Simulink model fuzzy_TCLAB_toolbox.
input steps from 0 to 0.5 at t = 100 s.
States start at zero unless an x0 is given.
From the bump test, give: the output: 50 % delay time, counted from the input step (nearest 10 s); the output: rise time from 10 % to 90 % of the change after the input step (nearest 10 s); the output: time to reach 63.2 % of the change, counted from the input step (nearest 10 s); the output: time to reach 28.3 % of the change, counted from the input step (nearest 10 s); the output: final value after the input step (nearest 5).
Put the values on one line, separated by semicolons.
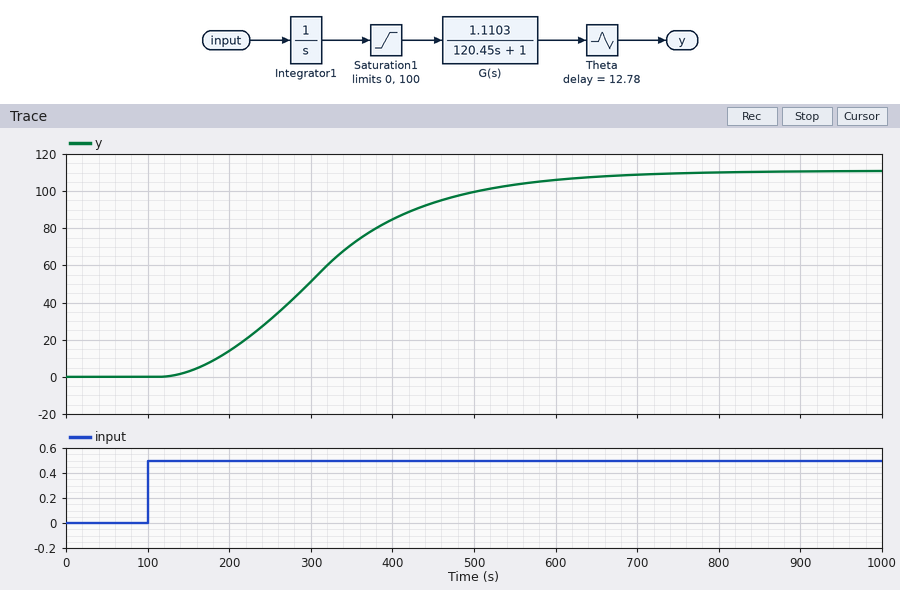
210 s; 310 s; 250 s; 150 s; 110
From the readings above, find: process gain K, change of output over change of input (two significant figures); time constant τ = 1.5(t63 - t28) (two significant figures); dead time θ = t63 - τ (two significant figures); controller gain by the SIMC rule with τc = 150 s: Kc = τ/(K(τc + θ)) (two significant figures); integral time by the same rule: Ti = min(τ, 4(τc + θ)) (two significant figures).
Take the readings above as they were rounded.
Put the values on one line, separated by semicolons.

220; 150 s; 100 s; 0.0027; 150 s
